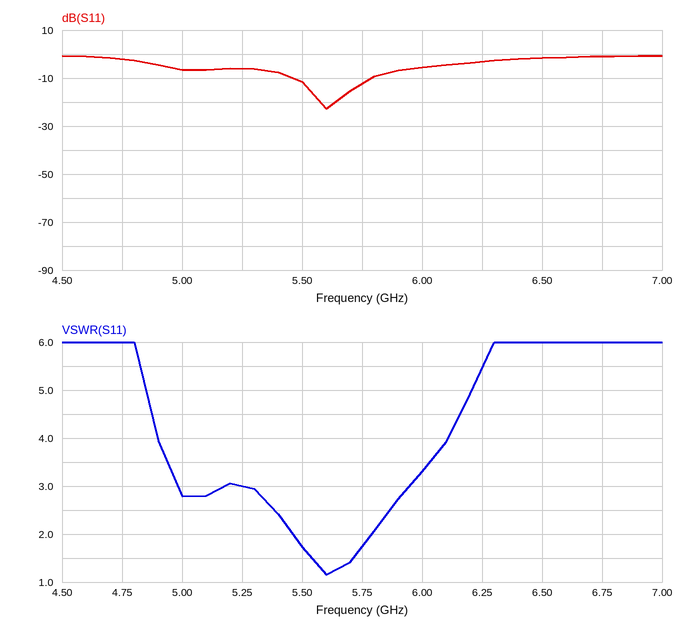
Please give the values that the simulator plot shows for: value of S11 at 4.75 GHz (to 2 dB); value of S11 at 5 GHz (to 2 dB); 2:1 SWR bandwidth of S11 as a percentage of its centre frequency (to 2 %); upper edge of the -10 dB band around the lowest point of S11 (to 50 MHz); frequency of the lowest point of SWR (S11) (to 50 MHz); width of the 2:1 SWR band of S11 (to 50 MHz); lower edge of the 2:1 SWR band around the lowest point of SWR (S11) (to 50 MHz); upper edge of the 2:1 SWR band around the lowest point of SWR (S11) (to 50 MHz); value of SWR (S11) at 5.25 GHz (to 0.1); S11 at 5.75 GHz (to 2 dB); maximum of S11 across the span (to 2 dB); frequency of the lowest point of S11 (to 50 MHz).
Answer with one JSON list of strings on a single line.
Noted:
["-2 dB", "-6 dB", "6 %", "5.80 GHz", "5.60 GHz", "350 MHz", "5.45 GHz", "5.80 GHz", "3.0", "-12 dB", "0 dB", "5.60 GHz"]
